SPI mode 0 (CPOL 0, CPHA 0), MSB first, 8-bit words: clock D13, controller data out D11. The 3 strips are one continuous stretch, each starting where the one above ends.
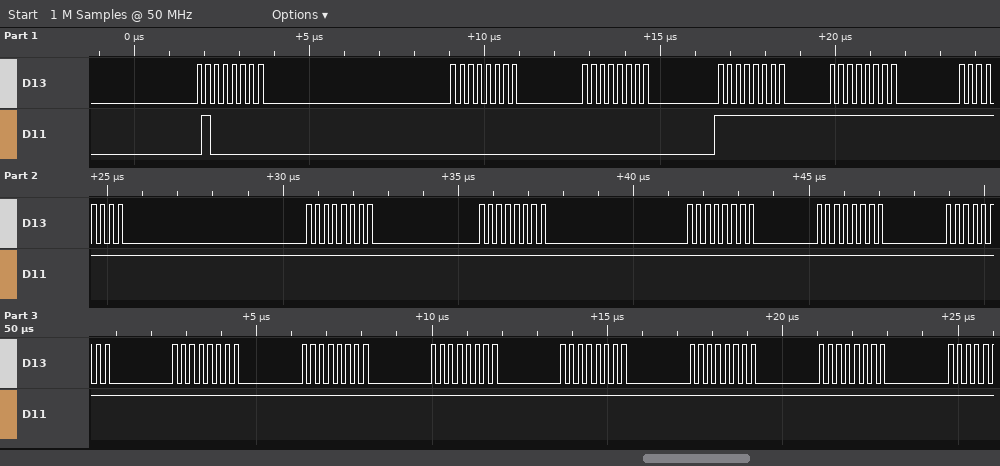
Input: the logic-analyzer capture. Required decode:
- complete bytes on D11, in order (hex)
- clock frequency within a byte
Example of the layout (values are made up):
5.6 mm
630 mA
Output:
40 00 00 FF FF FF FF FF FF FF FF FF FF FF FF FF FF
4 MHz
